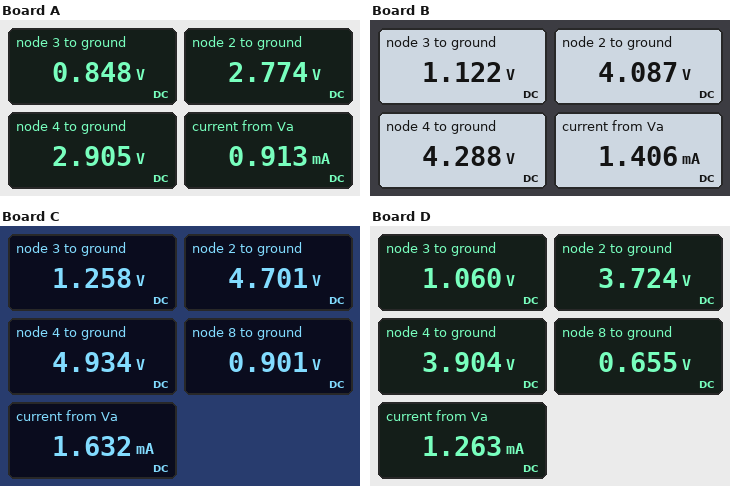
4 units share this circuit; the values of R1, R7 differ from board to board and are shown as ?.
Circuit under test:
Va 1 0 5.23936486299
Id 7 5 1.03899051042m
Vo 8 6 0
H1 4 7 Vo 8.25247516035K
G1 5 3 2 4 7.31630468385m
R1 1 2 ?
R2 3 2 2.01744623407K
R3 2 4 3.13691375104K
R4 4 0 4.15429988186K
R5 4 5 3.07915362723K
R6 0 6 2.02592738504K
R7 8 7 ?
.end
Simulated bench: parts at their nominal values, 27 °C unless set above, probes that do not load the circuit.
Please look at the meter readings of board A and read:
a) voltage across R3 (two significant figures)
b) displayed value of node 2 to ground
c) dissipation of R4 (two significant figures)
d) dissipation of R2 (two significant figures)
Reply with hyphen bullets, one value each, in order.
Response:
- 130 mV
- 2.774 V
- 2.0 mW
- 1.8 mW
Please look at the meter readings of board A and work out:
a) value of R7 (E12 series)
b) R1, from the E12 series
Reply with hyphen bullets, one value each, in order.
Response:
- 3.3 kΩ
- 2.7 kΩ
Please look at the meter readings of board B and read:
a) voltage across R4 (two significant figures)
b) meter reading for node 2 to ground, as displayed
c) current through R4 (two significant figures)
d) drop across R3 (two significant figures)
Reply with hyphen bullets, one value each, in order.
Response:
- 4.3 V
- 4.087 V
- 1.0 mA
- 200 mV
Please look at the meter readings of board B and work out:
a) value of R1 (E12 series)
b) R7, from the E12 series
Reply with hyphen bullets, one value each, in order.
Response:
- 820 Ω
- 1.2 kΩ
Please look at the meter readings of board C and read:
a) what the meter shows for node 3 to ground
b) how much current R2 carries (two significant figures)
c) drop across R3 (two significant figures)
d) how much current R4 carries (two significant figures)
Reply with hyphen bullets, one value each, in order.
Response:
- 1.258 V
- 1.7 mA
- 230 mV
- 1.2 mA
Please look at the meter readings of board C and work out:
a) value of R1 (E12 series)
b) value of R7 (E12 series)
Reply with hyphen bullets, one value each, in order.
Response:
- 330 Ω
- 820 Ω
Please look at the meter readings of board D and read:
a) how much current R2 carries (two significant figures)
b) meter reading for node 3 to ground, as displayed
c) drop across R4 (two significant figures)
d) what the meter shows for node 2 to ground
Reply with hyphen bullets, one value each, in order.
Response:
- 1.3 mA
- 1.060 V
- 3.9 V
- 3.724 V
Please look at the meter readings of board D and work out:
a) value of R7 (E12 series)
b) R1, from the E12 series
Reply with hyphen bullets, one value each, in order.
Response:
- 1.8 kΩ
- 1.2 kΩ
